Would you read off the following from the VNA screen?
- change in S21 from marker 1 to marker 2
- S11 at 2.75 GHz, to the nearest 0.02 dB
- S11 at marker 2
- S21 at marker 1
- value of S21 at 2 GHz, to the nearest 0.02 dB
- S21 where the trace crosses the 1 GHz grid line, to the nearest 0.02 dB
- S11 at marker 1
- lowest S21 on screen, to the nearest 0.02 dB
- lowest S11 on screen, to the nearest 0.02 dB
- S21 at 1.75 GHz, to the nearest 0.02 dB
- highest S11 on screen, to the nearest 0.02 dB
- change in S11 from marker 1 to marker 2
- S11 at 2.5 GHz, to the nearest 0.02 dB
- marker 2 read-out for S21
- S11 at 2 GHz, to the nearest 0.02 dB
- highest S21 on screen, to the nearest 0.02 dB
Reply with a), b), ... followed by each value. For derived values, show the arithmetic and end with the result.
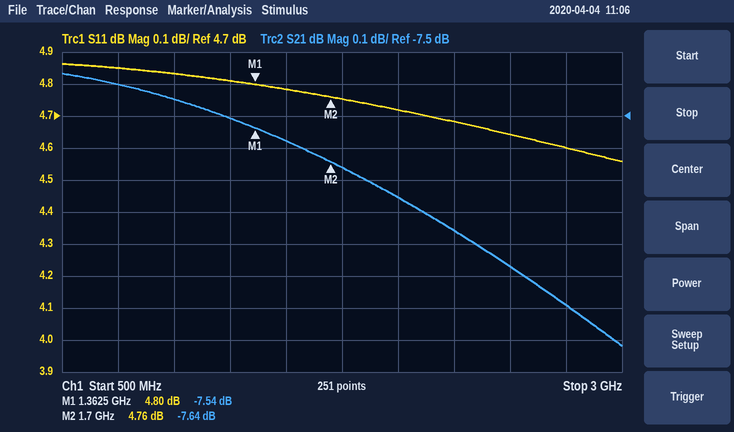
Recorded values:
a) -7.64 − (-7.54) = -0.10 dB
b) 4.60 dB
c) 4.76 dB
d) -7.54 dB
e) -7.76 dB
f) -7.44 dB
g) 4.80 dB
h) -8.22 dB
i) 4.56 dB
j) -7.66 dB
k) 4.86 dB
l) 4.76 − (4.8) = -0.04 dB
m) 4.64 dB
n) -7.64 dB
o) 4.72 dB
p) -7.36 dB
